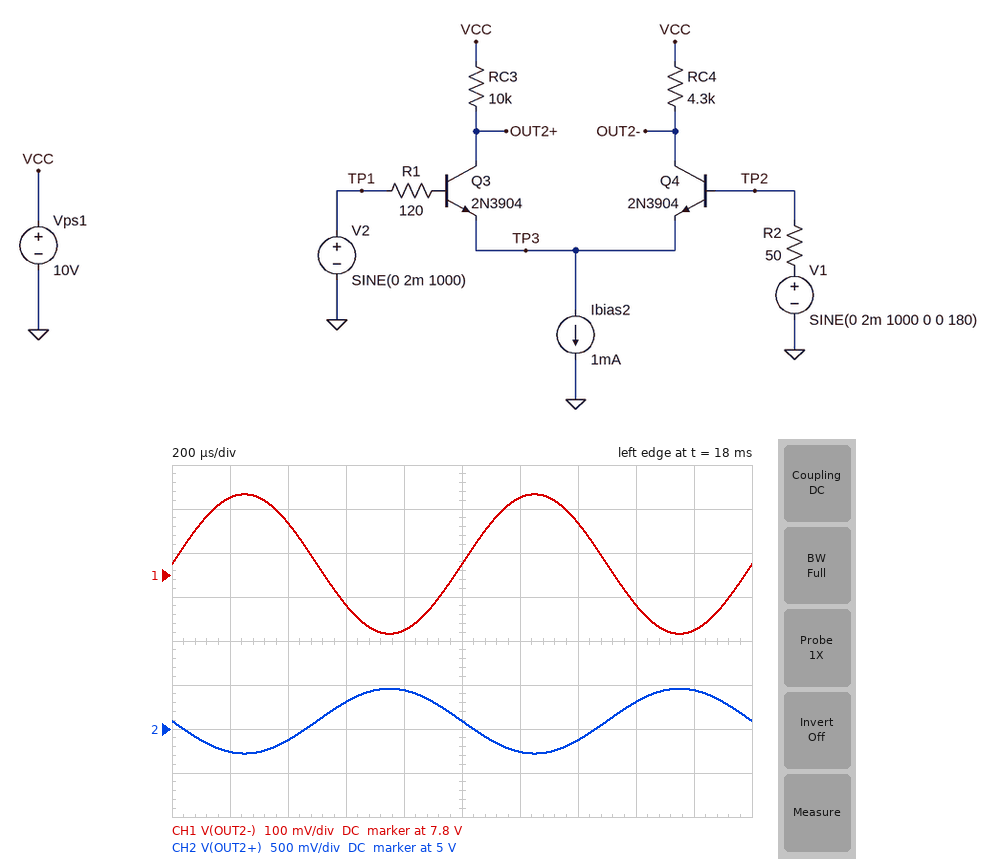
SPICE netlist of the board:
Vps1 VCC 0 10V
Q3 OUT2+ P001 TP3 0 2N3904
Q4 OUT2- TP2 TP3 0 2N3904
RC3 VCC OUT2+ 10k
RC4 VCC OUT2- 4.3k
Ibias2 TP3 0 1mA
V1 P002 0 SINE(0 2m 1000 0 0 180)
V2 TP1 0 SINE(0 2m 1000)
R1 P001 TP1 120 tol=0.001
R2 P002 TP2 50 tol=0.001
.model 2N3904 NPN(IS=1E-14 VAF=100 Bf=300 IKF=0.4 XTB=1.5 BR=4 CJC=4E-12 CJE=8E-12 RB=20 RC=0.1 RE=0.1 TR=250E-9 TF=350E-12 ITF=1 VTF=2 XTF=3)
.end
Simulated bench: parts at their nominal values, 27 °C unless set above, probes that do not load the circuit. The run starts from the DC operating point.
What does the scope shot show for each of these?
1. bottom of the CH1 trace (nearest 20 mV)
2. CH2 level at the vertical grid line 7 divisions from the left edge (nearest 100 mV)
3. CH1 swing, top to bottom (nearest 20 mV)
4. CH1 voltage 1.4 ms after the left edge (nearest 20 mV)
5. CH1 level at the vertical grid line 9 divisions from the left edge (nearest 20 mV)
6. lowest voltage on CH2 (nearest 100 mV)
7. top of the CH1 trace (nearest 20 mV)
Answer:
7.66 V
4.9 V
320 mV
7.92 V
7.68 V
4.7 V
7.98 V
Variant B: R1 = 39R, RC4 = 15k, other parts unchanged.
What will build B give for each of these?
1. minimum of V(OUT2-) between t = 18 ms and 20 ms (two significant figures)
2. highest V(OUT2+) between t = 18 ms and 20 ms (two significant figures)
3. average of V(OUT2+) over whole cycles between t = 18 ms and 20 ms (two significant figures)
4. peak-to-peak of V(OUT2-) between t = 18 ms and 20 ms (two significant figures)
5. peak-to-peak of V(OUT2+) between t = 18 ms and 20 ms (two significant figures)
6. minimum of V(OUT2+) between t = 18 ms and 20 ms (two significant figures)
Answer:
2.1 V
5.3 V
5.0 V
1.1 V
720 mV
4.6 V
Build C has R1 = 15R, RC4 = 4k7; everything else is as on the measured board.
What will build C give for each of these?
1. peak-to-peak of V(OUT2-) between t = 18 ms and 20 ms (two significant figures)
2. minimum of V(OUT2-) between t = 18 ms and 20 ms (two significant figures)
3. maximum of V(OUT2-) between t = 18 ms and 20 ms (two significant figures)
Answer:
350 mV
7.5 V
7.8 V
